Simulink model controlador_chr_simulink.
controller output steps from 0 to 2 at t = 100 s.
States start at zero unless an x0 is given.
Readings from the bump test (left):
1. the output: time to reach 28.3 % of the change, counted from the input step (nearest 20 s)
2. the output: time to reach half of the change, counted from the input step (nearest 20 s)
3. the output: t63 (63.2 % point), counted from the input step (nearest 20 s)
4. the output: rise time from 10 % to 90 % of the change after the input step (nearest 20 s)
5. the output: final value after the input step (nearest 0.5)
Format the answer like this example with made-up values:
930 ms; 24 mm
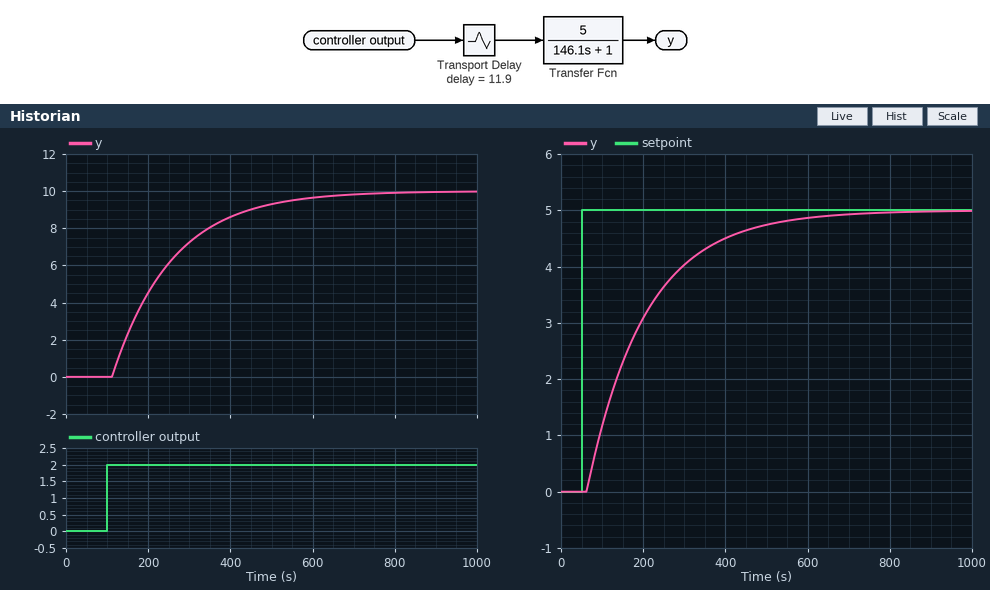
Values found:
60 s; 120 s; 160 s; 320 s; 10.0
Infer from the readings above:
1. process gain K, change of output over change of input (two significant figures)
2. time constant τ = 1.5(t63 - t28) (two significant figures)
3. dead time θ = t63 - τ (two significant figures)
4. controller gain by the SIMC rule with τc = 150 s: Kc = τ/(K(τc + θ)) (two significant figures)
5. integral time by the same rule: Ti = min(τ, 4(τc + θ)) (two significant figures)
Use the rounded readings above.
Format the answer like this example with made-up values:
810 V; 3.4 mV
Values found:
5.0; 150 s; 10 s; 0.19; 150 s
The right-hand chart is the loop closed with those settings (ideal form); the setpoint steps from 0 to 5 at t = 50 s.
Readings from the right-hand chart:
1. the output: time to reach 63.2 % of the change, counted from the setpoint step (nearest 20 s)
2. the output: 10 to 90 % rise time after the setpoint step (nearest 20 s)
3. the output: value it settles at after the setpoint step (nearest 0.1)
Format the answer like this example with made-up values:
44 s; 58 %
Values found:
160 s; 320 s; 5.0
